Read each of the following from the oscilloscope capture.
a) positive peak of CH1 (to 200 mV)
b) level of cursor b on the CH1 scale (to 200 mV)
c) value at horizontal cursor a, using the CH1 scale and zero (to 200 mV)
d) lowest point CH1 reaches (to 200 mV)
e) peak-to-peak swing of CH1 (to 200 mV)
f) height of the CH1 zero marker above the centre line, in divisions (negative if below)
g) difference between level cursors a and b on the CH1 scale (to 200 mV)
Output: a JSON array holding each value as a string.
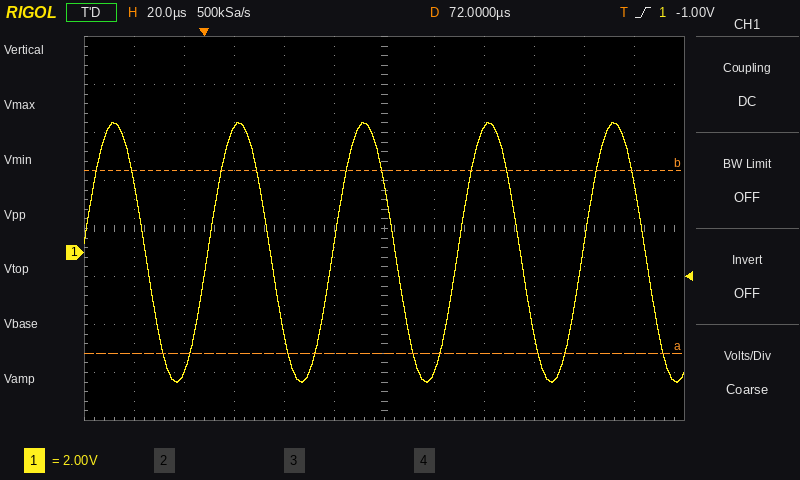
["5.4 V", "3.4 V", "-4.2 V", "-5.4 V", "10.8 V", "-0.5 div", "7.6 V"]
